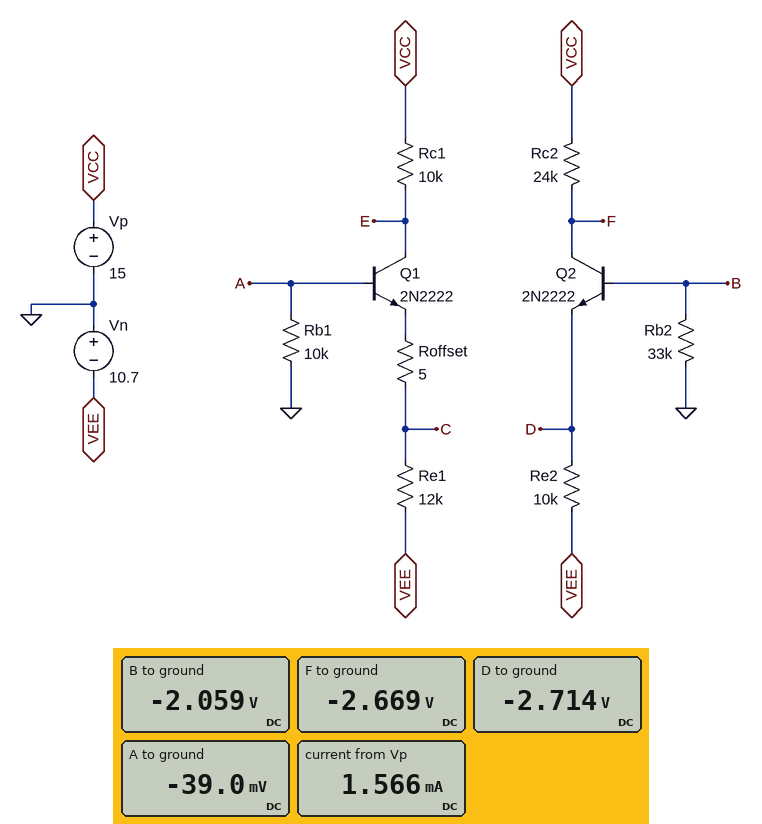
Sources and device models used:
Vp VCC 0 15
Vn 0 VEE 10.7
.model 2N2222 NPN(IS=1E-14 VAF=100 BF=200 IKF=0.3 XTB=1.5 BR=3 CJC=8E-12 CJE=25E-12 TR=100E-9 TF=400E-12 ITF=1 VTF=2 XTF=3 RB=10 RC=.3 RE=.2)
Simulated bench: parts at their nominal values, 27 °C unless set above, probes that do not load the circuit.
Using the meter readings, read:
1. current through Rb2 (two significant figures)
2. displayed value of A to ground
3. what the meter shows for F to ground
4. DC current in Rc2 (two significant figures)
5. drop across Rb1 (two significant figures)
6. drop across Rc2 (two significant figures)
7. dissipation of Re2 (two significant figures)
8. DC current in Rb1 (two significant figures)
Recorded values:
62 µA
-39.0 mV
-2.669 V
740 µA
39 mV
18 V
6.4 mW
3.9 µA
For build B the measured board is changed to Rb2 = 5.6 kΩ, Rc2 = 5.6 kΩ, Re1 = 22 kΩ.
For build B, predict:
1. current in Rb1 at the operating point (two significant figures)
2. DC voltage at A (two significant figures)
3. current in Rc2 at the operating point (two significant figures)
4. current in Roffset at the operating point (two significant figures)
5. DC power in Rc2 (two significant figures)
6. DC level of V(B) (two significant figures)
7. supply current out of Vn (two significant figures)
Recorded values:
2.1 µA
-21 mV
1.0 mA
460 µA
5.6 mW
-26 mV
1.5 mA
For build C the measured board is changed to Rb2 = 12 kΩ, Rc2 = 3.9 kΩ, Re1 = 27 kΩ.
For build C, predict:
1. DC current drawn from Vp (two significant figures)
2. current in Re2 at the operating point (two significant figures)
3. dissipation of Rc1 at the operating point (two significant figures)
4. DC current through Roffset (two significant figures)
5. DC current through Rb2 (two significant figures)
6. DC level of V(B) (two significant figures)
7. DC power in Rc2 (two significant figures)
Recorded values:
1.4 mA
1.0 mA
1.4 mW
370 µA
4.5 µA
-54 mV
3.9 mW
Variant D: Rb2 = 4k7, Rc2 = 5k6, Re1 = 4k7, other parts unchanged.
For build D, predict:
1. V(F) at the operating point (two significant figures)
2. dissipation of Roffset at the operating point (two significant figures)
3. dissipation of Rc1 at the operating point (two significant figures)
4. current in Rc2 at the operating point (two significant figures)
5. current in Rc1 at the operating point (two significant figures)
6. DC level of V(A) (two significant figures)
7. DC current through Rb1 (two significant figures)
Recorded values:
9.4 V
17 µW
29 mW
1.0 mA
1.7 mA
-1.4 V
140 µA
